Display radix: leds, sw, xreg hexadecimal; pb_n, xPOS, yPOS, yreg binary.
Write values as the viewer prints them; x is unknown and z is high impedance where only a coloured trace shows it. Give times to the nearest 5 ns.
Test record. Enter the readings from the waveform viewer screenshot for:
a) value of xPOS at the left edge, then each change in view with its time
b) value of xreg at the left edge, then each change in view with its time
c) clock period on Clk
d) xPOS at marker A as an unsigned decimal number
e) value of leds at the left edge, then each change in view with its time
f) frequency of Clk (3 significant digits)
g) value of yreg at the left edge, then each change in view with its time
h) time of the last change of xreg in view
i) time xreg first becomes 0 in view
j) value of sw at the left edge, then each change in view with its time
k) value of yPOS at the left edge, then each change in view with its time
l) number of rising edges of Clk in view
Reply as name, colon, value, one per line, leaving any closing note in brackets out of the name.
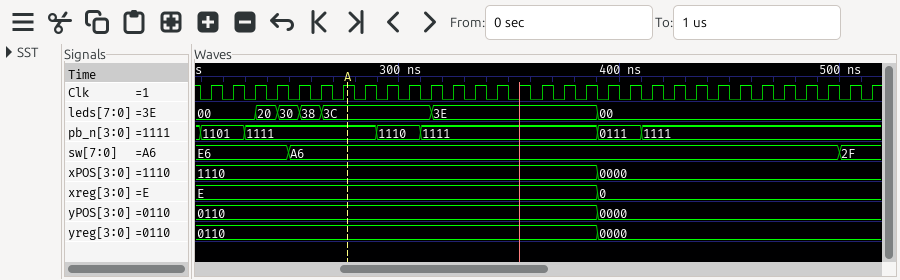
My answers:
value of xPOS at the left edge, then each change in view with its time: 1110, 0000 at 390 ns
value of xreg at the left edge, then each change in view with its time: E, 0 at 390 ns
clock period on Clk: 10 ns
xPOS at marker A as an unsigned decimal number: 14
value of leds at the left edge, then each change in view with its time: 00, 20 at 235 ns, 30 at 245 ns, 38 at 255 ns, 3C at 265 ns, 3E at 315 ns, 00 at 390 ns
frequency of Clk: 100 MHz
value of yreg at the left edge, then each change in view with its time: 0110, 0000 at 390 ns
time of the last change of xreg in view: 390 ns
time xreg first becomes 0 in view: 390 ns
value of sw at the left edge, then each change in view with its time: E6, A6 at 250 ns, 2F at 500 ns
value of yPOS at the left edge, then each change in view with its time: 0110, 0000 at 390 ns
number of rising edges of Clk in view: 31
